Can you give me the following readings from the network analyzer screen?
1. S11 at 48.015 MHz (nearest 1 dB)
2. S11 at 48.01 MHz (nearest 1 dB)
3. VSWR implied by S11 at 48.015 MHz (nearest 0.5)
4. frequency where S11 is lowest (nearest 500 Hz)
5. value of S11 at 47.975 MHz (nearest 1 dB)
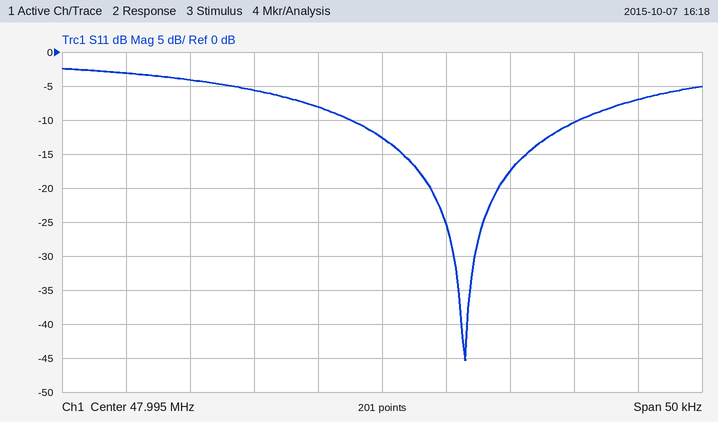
-7 dB
-10 dB
2.5
48.0015 MHz
-3 dB
